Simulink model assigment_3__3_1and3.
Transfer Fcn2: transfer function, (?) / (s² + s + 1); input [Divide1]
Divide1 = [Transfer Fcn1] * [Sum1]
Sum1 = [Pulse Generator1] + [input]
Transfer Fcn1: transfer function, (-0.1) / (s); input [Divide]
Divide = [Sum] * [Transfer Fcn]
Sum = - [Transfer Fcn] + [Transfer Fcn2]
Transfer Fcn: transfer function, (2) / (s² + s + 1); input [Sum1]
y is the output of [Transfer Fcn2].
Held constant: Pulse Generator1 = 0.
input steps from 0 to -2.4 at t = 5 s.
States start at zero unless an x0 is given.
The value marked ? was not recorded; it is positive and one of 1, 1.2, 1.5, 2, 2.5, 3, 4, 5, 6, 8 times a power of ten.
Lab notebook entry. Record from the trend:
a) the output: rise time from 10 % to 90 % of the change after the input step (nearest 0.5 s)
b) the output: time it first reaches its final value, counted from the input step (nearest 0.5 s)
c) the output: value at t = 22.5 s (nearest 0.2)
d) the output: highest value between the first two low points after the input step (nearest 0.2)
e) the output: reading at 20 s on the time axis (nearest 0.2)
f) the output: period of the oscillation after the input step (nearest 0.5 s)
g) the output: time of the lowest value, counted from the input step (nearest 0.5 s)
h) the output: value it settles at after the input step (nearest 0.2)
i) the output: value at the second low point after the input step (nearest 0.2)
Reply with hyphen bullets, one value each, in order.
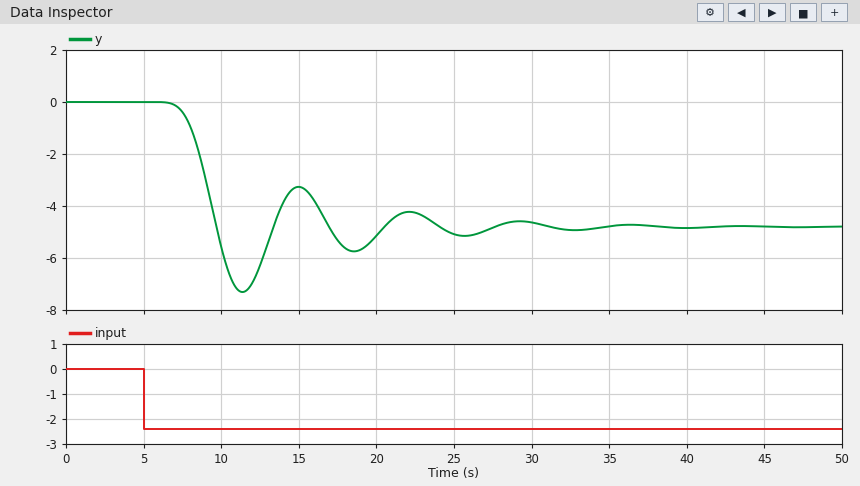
- 2.0 s
- 4.5 s
- -4.2
- -3.2
- -5.2
- 7.0 s
- 6.5 s
- -4.8
- -5.8
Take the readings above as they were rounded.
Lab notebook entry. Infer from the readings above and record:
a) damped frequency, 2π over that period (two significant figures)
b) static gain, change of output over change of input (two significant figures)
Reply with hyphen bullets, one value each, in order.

- 0.90 rad/s
- 2.0
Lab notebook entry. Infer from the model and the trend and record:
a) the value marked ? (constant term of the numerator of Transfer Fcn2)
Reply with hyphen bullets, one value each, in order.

- 0.5
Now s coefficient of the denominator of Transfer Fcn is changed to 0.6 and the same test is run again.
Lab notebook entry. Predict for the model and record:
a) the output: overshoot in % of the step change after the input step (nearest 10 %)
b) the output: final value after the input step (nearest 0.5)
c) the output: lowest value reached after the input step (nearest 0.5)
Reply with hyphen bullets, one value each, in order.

- 90 %
- -5.0
- -9.0
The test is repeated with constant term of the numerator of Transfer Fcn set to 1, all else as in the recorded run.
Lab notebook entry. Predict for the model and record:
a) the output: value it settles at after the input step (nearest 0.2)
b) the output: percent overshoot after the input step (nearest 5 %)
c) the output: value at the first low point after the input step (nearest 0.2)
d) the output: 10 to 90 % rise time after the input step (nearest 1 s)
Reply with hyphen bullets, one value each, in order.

- -2.4
- 10 %
- -2.6
- 3 s
